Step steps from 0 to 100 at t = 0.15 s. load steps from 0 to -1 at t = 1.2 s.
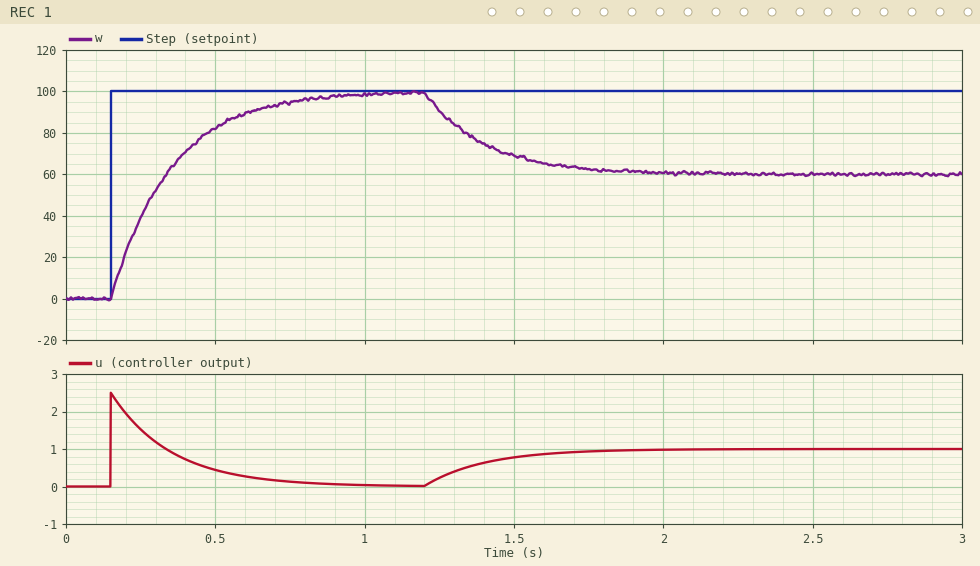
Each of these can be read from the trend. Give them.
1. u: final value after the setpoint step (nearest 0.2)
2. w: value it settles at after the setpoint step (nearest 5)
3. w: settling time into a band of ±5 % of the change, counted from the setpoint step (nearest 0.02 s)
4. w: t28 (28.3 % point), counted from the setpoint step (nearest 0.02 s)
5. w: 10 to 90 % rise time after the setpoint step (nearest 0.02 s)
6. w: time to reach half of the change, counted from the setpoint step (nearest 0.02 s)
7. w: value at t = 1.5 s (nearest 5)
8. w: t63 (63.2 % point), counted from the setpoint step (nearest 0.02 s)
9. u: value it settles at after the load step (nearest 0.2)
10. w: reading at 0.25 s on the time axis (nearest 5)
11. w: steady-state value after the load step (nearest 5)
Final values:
0.0
100
0.60 s
0.06 s
0.44 s
0.14 s
70
0.20 s
1.0
40
60
